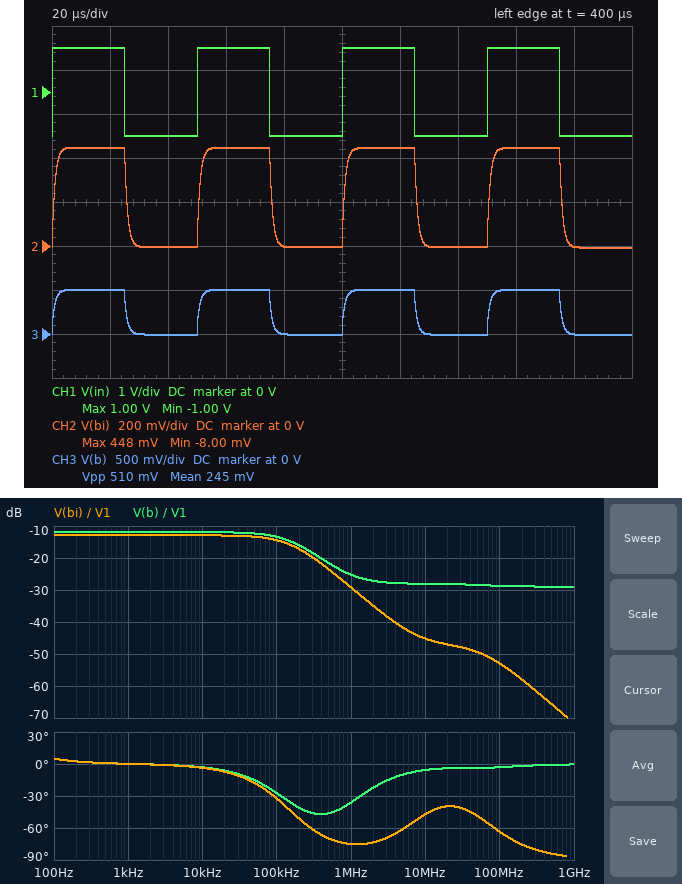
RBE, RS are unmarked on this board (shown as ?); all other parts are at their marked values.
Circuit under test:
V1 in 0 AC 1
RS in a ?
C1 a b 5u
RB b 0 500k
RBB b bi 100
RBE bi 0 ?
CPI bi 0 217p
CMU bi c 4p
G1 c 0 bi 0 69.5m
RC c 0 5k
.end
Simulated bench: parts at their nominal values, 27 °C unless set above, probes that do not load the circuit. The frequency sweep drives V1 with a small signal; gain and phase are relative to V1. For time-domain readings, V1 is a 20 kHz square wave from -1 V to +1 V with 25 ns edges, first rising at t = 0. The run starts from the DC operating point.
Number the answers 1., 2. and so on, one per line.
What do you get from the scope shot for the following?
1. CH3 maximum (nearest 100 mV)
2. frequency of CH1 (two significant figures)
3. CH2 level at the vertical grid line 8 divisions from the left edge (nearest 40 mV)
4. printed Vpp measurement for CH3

1. 500 mV
2. 20 kHz
3. 440 mV
4. 510 mV
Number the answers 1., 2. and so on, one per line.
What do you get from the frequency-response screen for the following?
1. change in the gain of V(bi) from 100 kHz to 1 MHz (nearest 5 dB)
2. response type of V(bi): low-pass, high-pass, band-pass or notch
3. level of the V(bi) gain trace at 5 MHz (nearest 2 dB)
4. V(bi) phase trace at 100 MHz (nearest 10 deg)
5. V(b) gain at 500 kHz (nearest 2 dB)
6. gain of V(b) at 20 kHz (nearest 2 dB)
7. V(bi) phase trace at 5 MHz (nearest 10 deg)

1. -15 dB
2. low-pass
3. -42 dB
4. -60 deg
5. -22 dB
6. -12 dB
7. -60 deg
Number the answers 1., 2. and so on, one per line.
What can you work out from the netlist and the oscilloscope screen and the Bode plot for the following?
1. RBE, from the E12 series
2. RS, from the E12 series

1. 820 Ω
2. 2.7 kΩ
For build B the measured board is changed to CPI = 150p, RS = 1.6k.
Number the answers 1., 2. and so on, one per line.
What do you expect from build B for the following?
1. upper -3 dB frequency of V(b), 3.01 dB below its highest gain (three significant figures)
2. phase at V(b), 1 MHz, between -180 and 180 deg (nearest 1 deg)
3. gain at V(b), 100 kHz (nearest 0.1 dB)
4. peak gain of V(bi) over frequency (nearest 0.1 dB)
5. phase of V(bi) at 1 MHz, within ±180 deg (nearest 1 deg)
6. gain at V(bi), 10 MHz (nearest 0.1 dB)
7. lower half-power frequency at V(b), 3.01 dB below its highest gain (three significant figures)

1. 189 kHz
2. -35 deg
3. -9.9 dB
4. -9.8 dB
5. -73 deg
6. -40.5 dB
7. 12.6 Hz
